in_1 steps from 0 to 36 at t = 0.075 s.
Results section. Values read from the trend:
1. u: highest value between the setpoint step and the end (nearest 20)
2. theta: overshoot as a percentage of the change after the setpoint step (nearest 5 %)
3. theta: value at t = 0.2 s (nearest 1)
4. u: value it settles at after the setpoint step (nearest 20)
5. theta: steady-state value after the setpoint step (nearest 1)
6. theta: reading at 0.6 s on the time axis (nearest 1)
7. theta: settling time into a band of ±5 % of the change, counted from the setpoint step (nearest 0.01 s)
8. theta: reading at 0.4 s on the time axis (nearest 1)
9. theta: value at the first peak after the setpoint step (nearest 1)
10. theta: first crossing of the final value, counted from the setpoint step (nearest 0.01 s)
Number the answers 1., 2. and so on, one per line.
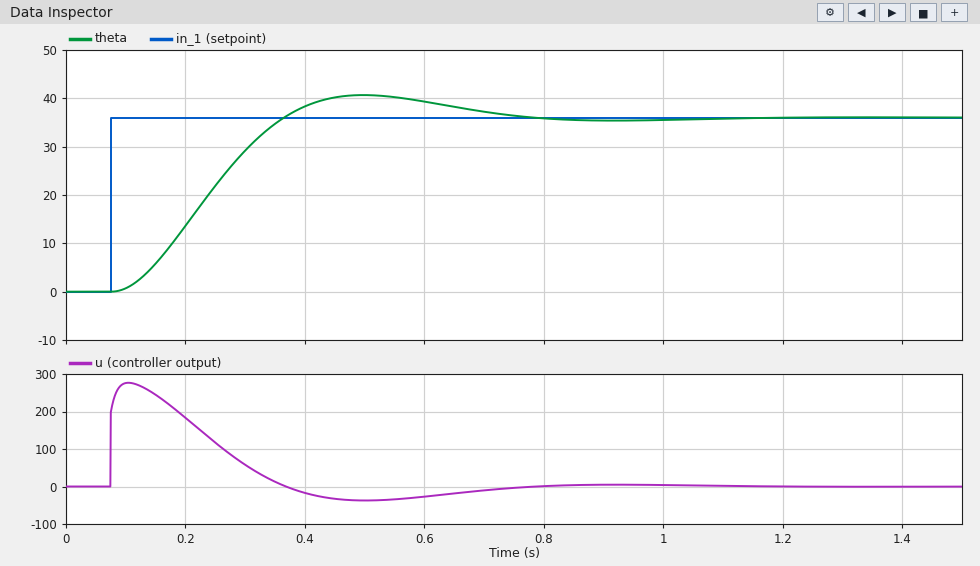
1. 280
2. 15 %
3. 14
4. 0
5. 36
6. 39
7. 0.60 s
8. 38
9. 41
10. 0.29 s
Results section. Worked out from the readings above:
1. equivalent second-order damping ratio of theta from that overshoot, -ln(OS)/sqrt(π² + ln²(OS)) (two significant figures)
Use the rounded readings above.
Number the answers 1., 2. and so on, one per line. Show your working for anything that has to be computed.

1. ln(0.15) = -1.897; 1.897 / sqrt(9.870 + 3.599) = 0.52
